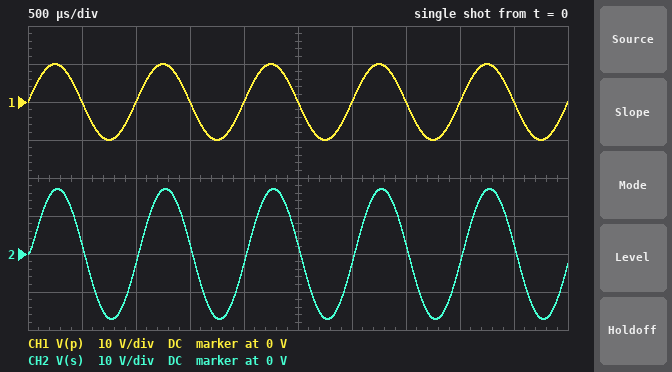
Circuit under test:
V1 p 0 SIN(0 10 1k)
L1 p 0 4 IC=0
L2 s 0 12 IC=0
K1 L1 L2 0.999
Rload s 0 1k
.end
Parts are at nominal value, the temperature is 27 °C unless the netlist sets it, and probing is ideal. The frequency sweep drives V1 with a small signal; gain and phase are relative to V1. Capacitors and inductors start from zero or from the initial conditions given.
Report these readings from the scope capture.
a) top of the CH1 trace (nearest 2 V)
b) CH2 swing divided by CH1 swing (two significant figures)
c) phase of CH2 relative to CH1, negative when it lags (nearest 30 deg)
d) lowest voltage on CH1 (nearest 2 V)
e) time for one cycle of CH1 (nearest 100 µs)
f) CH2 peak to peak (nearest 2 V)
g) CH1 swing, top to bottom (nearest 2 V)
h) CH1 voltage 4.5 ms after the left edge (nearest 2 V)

10 V
1.7
0 deg
-10 V
1.0 ms
34 V
20 V
0 V
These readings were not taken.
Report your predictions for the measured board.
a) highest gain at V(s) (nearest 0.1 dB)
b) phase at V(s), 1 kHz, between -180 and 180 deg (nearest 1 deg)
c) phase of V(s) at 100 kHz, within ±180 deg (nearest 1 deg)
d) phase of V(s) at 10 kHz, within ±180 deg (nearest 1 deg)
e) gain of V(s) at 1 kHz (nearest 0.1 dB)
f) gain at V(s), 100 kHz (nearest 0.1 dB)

4.8 dB
-9 deg
-86 deg
-56 deg
4.7 dB
-18.8 dB
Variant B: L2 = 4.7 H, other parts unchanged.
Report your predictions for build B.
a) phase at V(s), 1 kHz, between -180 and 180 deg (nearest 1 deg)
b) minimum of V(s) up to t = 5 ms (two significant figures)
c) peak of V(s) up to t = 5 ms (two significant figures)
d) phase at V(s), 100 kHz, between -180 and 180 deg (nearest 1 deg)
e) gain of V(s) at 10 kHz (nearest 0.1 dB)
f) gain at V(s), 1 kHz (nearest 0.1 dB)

-3 deg
-11 V
11 V
-80 deg
-0.6 dB
0.7 dB
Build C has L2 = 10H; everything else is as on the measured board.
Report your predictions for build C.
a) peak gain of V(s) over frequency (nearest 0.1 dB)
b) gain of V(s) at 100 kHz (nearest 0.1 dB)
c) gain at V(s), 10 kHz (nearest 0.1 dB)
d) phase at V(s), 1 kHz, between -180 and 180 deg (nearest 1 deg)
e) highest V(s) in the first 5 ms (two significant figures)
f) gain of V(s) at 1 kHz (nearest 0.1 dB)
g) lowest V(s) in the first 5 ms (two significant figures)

4.0 dB
-18.0 dB
-0.1 dB
-7 deg
16 V
3.9 dB
-16 V
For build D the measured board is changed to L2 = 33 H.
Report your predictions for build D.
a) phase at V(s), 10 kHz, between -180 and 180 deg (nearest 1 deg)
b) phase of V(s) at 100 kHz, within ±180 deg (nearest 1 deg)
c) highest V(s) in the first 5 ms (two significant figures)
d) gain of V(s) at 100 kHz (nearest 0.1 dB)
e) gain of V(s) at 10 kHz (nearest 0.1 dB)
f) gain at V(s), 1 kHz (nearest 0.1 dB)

-76 deg
-89 deg
27 V
-23.2 dB
-3.4 dB
8.5 dB
